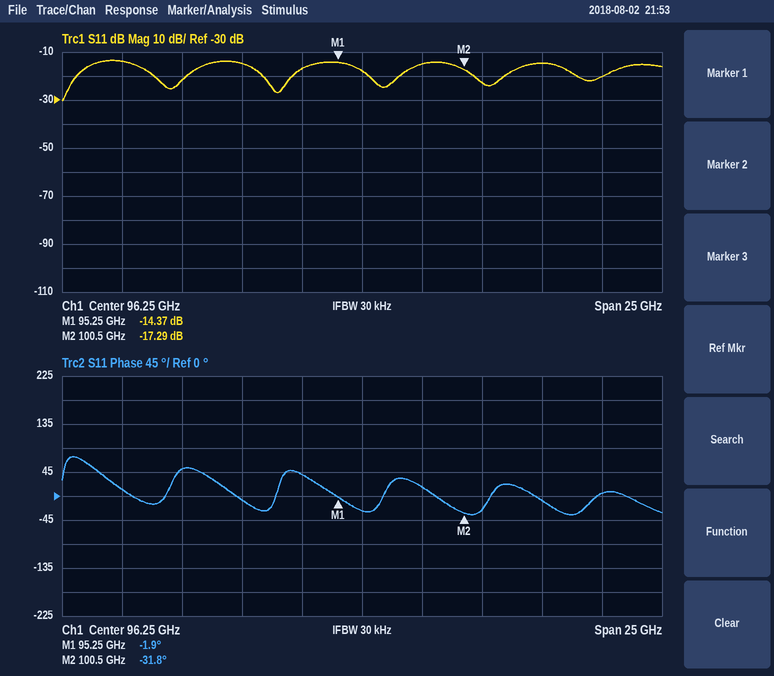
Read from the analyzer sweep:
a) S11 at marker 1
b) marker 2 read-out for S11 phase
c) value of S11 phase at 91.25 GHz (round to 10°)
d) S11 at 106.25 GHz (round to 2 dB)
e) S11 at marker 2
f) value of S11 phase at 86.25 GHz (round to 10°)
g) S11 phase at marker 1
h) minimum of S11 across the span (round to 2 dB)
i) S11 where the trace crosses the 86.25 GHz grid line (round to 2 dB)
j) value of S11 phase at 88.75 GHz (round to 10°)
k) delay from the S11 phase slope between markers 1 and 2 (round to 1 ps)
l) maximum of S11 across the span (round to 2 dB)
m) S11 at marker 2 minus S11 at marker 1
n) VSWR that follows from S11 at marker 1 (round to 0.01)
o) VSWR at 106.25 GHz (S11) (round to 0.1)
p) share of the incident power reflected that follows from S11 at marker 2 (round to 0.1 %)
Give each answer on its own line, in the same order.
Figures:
-14.37 dB
-31.8°
-10°
-20 dB
-17.29 dB
10°
-1.9°
-30 dB
-14 dB
50°
16 ps
-14 dB
-2.92 dB
1.47
1.2
1.9 %
